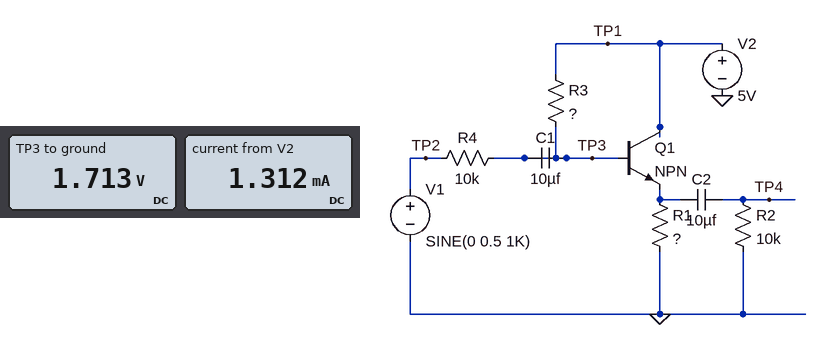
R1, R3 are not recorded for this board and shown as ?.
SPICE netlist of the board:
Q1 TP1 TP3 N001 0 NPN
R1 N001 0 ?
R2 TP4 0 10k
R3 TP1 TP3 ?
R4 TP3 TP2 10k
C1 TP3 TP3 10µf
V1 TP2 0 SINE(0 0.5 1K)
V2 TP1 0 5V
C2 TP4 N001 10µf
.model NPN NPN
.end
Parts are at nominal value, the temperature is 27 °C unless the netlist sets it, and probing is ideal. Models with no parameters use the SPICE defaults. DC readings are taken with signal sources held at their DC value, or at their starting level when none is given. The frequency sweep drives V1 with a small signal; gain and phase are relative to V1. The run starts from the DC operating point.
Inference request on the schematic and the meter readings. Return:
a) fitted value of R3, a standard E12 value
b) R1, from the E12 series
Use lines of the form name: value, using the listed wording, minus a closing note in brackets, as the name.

fitted value of R3, a standard E12 value: 18 kΩ
R1, from the E12 series: 820 Ω
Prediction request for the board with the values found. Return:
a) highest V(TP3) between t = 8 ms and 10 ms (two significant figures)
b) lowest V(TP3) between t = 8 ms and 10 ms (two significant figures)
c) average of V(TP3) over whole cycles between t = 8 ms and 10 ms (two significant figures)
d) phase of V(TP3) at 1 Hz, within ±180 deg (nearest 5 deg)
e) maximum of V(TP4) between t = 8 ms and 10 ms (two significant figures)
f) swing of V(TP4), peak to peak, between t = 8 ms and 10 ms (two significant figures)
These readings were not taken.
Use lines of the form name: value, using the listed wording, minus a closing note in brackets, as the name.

highest V(TP3) between t = 8 ms and 10 ms: 2.0 V
lowest V(TP3) between t = 8 ms and 10 ms: 1.4 V
average of V(TP3) over whole cycles between t = 8 ms and 10 ms: 1.7 V
phase of V(TP3) at 1 Hz, within ±180 deg: 0 deg
maximum of V(TP4) between t = 8 ms and 10 ms: 290 mV
swing of V(TP4), peak to peak, between t = 8 ms and 10 ms: 580 mV
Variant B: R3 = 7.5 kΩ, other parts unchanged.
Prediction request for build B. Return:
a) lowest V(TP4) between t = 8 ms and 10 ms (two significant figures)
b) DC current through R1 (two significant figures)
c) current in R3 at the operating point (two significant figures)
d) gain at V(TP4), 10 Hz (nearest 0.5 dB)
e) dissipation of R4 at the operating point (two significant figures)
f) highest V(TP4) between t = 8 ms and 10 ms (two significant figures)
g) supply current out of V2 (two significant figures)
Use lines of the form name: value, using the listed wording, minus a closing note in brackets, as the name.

lowest V(TP4) between t = 8 ms and 10 ms: -200 mV
DC current through R1: 2.4 mA
current in R3 at the operating point: 300 µA
gain at V(TP4), 10 Hz: -8.0 dB
dissipation of R4 at the operating point: 760 µW
highest V(TP4) between t = 8 ms and 10 ms: 200 mV
supply current out of V2: 2.7 mA
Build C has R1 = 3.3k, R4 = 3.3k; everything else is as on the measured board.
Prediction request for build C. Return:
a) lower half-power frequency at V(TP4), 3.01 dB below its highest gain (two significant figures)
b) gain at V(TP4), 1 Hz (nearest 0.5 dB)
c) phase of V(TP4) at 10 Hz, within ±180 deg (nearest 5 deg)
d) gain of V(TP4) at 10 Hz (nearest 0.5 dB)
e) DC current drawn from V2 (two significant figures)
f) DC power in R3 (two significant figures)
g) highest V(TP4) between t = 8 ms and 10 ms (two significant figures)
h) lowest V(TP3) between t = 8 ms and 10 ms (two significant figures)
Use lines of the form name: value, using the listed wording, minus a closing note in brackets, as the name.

lower half-power frequency at V(TP4), 3.01 dB below its highest gain: 1.5 Hz
gain at V(TP4), 1 Hz: -9.5 dB
phase of V(TP4) at 10 Hz, within ±180 deg: 10 deg
gain of V(TP4) at 10 Hz: -4.5 dB
DC current drawn from V2: 260 µA
DC power in R3: 990 µW
highest V(TP4) between t = 8 ms and 10 ms: 360 mV
lowest V(TP3) between t = 8 ms and 10 ms: 350 mV
